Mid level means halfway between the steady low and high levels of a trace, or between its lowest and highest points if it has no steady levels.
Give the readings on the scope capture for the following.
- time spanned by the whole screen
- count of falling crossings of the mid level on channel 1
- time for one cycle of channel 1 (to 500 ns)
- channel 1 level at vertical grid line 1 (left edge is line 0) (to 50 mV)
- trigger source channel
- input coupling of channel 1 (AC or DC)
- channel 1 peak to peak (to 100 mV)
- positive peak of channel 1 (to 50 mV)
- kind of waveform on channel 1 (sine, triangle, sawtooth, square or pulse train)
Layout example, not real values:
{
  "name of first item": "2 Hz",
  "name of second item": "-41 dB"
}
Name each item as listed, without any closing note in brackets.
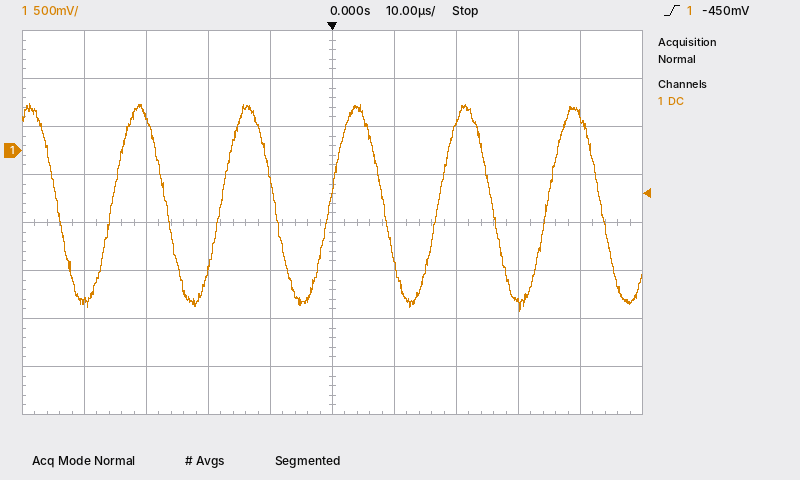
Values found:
{
  "time spanned by the whole screen": "100 µs",
  "count of falling crossings of the mid level on channel 1": "6",
  "time for one cycle of channel 1": "17.5 µs",
  "channel 1 level at vertical grid line 1 (left edge is line 0)": "-1.55 V",
  "trigger source channel": "channel 1",
  "input coupling of channel 1": "DC",
  "channel 1 peak to peak": "2.20 V",
  "positive peak of channel 1": "500 mV",
  "kind of waveform on channel 1": "sine"
}
